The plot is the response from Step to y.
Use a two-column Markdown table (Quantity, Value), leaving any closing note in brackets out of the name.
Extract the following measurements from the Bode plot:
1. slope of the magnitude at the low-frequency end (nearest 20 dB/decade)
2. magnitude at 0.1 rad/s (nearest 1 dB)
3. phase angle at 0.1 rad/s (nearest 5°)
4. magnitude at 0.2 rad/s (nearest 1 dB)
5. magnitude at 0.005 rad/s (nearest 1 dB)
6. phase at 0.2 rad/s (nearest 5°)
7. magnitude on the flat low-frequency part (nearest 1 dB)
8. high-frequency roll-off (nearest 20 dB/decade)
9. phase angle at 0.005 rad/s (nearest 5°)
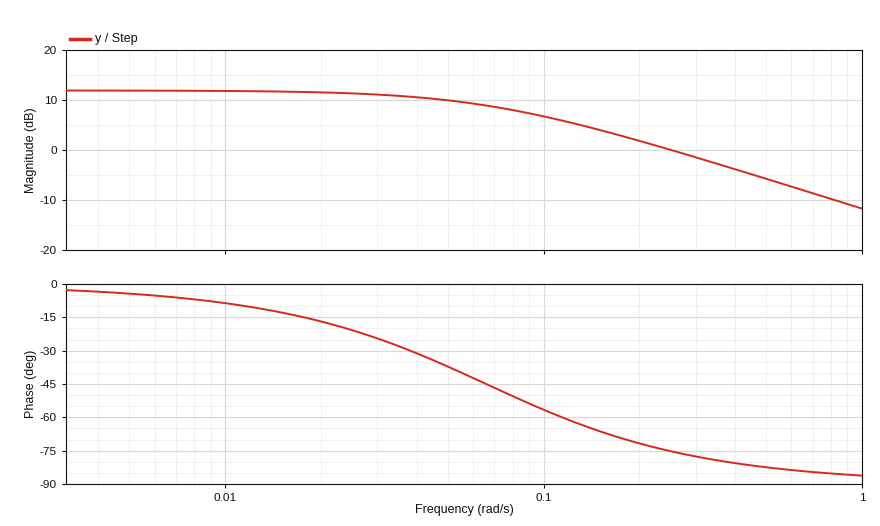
| Quantity | Value |
|---|---|
| slope of the magnitude at the low-frequency end | 0 dB/decade |
| magnitude at 0.1 rad/s | 7 dB |
| phase angle at 0.1 rad/s | -55° |
| magnitude at 0.2 rad/s | 2 dB |
| magnitude at 0.005 rad/s | 12 dB |
| phase at 0.2 rad/s | -70° |
| magnitude on the flat low-frequency part | 12 dB |
| high-frequency roll-off | -20 dB/decade |
| phase angle at 0.005 rad/s | -5° |
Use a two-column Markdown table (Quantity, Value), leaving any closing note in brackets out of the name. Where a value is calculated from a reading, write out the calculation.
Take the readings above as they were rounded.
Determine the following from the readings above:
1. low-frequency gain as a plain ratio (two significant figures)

| Quantity | Value |
|---|---|
| low-frequency gain as a plain ratio | 10^(12 / 20) = 4.0 |
